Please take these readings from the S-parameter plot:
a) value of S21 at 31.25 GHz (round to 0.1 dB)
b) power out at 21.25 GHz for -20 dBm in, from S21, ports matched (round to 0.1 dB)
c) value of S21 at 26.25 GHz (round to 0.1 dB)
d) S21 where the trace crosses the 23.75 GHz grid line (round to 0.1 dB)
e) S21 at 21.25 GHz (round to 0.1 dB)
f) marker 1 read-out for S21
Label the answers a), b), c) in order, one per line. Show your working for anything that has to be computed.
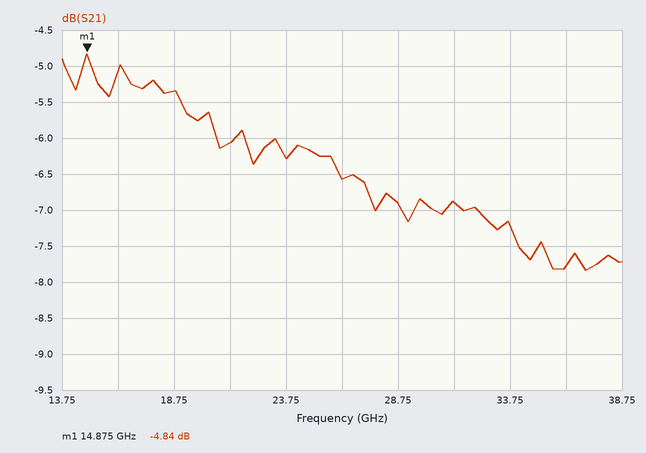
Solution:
a) -6.9 dB
b) -20 dBm + (-6.1 dB) = -26.1 dBm
c) -6.6 dB
d) -6.3 dB
e) -6.1 dB
f) -4.84 dB
